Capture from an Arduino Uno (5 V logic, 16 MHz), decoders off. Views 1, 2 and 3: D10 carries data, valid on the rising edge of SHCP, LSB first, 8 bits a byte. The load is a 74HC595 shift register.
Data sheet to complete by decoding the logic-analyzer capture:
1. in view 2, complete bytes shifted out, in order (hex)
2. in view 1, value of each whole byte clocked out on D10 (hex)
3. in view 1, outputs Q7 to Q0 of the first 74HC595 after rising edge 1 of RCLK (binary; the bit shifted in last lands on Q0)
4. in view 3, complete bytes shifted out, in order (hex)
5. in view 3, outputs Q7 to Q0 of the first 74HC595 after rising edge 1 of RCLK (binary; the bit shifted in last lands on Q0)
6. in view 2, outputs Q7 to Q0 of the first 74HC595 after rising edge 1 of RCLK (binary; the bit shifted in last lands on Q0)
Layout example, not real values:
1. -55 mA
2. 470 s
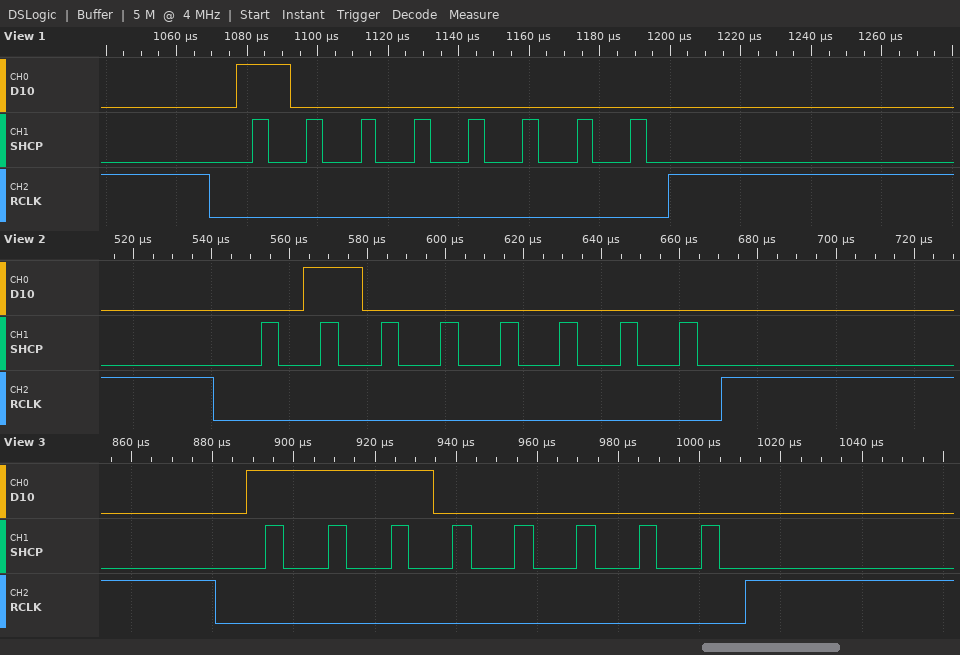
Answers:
1. 02
2. 01
3. 10000000
4. 07
5. 11100000
6. 01000000
